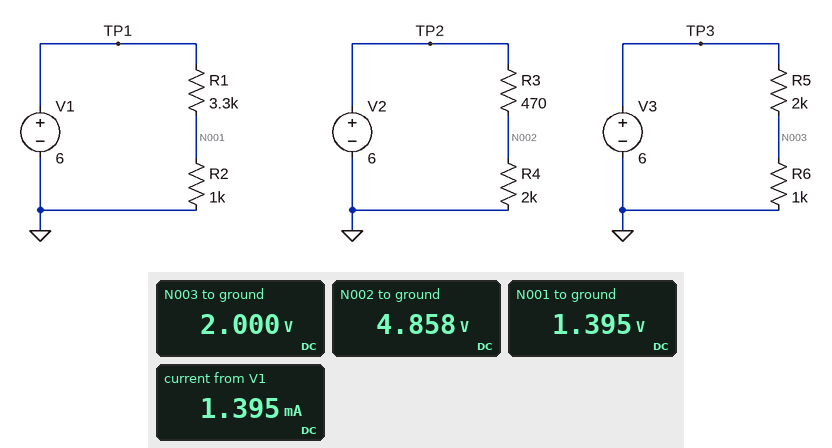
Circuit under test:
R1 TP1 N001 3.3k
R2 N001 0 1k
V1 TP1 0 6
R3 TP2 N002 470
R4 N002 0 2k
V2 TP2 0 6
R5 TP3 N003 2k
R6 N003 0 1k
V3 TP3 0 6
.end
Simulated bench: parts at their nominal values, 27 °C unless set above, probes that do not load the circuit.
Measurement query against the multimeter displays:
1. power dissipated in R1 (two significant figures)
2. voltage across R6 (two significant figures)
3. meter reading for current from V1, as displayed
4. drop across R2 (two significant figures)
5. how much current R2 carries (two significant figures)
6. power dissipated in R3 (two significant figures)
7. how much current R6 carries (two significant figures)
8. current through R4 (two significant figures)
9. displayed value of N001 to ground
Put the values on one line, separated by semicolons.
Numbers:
6.4 mW; 2.0 V; 1.395 mA; 1.4 V; 1.4 mA; 2.8 mW; 2.0 mA; 2.4 mA; 1.395 V
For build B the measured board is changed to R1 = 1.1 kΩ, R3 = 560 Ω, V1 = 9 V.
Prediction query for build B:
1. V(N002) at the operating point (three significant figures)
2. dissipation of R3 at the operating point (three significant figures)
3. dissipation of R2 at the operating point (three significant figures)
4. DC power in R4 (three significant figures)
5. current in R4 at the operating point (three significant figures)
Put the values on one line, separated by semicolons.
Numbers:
4.69 V; 3.08 mW; 18.4 mW; 11.0 mW; 2.34 mA
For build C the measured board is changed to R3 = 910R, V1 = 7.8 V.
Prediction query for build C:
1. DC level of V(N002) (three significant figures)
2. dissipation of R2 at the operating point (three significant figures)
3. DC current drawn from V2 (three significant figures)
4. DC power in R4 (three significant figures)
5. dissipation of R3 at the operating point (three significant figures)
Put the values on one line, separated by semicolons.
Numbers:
4.12 V; 3.29 mW; 2.06 mA; 8.50 mW; 3.87 mW
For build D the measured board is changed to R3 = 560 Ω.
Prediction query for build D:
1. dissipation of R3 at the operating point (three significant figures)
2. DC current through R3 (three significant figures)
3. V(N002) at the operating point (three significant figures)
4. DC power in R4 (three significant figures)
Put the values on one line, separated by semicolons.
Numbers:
3.08 mW; 2.34 mA; 4.69 V; 11.0 mW
